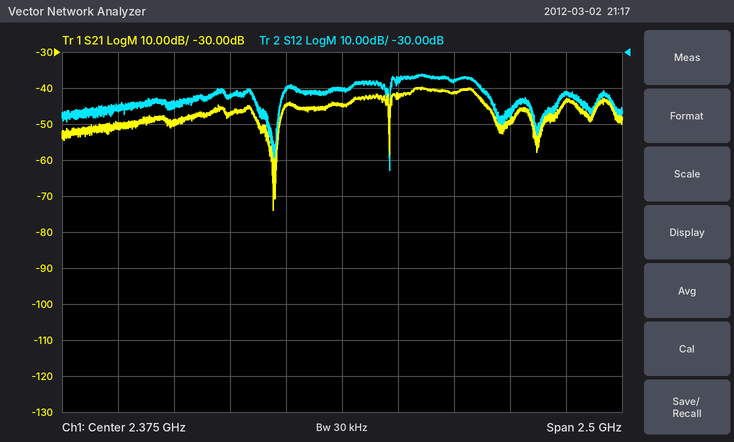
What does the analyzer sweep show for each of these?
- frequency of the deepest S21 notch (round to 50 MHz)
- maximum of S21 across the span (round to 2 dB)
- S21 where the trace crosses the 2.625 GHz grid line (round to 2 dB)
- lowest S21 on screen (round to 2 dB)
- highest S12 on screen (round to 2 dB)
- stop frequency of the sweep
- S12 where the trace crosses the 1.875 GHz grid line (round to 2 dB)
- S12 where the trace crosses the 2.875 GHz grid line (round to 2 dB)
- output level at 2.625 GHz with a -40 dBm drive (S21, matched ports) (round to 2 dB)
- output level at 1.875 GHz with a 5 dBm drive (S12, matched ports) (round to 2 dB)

2.05 GHz
-40 dB
-42 dB
-74 dB
-36 dB
3.625 GHz
-42 dB
-38 dB
-82 dBm
-38 dBm
